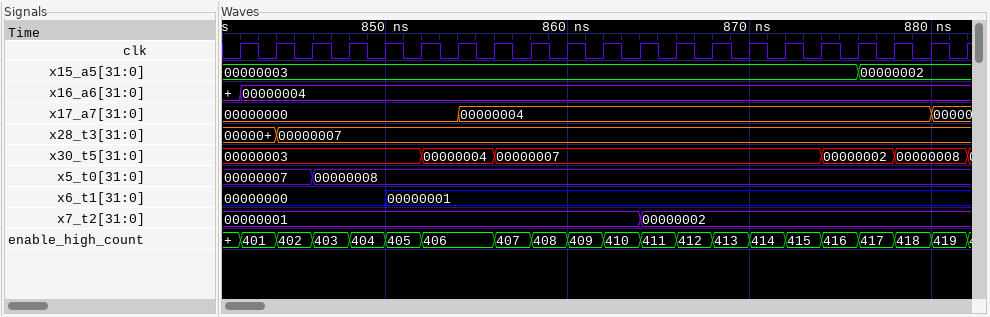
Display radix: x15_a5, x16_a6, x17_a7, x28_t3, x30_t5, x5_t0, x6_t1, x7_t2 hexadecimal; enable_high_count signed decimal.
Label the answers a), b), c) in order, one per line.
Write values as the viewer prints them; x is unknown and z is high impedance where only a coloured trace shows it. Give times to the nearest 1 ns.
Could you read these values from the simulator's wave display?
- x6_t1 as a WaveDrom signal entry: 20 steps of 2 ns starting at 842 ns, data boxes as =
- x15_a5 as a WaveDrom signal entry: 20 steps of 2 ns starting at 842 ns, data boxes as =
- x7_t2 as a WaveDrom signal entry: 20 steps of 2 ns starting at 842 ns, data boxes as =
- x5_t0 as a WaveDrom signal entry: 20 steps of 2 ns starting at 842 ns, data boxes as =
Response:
a) {name: 'x6_t1', wave: '=...=...............', data: '00000000 00000001'}
b) {name: 'x15_a5', wave: '=................=..', data: '00000003 00000002'}
c) {name: 'x7_t2', wave: '=..........=........', data: '00000001 00000002'}
d) {name: 'x5_t0', wave: '=.=.................', data: '00000007 00000008'}
